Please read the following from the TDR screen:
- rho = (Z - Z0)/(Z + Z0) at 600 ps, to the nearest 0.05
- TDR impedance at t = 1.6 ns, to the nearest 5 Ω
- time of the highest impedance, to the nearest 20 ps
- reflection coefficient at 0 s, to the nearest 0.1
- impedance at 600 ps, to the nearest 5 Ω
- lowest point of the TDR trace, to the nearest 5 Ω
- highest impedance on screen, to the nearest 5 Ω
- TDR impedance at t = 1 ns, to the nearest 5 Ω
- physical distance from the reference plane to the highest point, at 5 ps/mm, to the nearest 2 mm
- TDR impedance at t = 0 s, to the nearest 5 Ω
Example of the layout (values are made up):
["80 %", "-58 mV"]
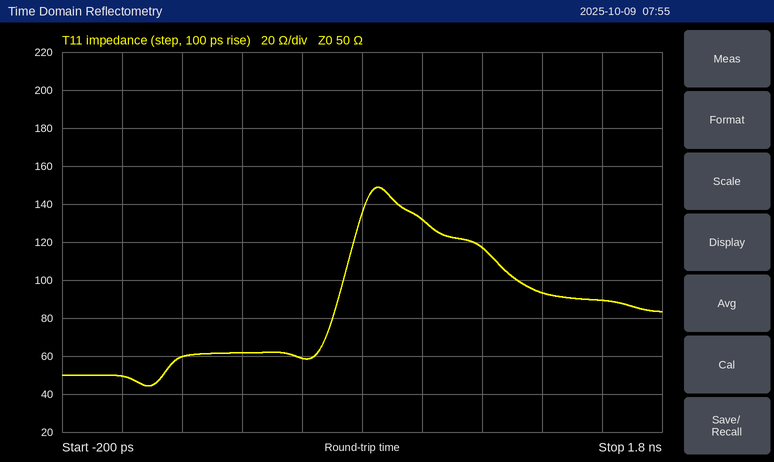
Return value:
["+0.10", "90 Ω", "860 ps", "0.0", "60 Ω", "45 Ω", "150 Ω", "130 Ω", "86 mm", "50 Ω"]
